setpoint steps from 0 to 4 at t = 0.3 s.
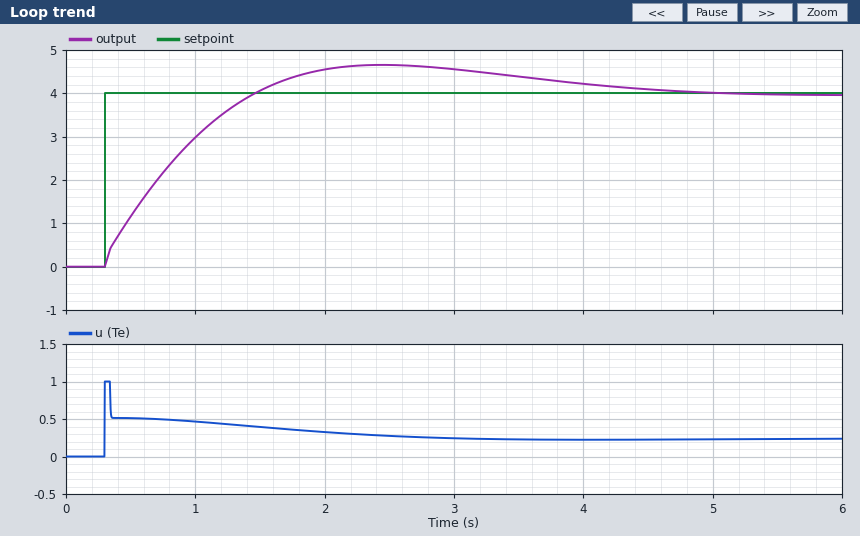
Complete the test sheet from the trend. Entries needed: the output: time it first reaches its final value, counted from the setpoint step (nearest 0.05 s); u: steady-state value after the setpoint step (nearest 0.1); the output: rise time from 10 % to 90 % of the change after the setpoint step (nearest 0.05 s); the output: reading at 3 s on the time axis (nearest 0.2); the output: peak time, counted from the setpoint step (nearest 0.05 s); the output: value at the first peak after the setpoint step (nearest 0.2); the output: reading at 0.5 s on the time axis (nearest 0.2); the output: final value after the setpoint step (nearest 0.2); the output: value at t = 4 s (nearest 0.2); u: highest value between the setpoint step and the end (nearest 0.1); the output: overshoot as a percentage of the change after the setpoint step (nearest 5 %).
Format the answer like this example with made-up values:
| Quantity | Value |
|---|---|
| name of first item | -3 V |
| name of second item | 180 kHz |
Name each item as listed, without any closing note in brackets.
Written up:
| Quantity | Value |
|---|---|
| the output: time it first reaches its final value, counted from the setpoint step | 1.15 s |
| u: steady-state value after the setpoint step | 0.2 |
| the output: rise time from 10 % to 90 % of the change after the setpoint step | 0.90 s |
| the output: reading at 3 s on the time axis | 4.6 |
| the output: peak time, counted from the setpoint step | 2.15 s |
| the output: value at the first peak after the setpoint step | 4.6 |
| the output: reading at 0.5 s on the time axis | 1.2 |
| the output: final value after the setpoint step | 4.0 |
| the output: value at t = 4 s | 4.2 |
| u: highest value between the setpoint step and the end | 1.0 |
| the output: overshoot as a percentage of the change after the setpoint step | 15 % |
